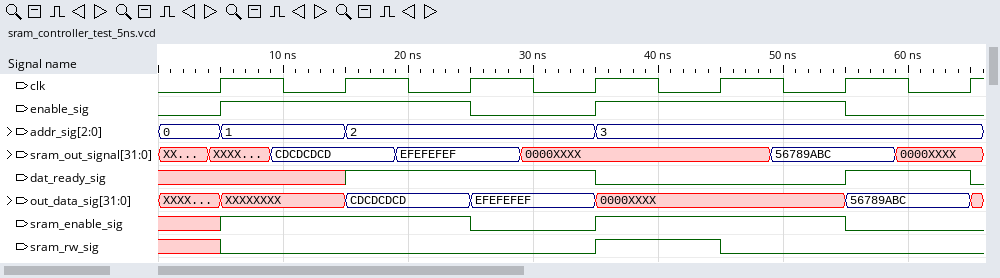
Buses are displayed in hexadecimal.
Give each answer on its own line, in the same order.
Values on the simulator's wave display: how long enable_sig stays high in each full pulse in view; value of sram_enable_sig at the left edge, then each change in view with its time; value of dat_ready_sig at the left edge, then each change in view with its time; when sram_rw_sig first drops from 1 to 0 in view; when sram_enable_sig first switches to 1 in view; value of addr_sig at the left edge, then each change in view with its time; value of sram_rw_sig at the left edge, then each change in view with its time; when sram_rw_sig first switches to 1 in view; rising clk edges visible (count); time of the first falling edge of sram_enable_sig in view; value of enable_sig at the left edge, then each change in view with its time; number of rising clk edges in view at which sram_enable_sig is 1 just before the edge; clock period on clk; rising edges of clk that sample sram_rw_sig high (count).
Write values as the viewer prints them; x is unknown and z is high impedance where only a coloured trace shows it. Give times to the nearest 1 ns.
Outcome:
20 ns, 20 ns
x, 1 at 5 ns, 0 at 25 ns, 1 at 35 ns, 0 at 55 ns
x, 1 at 15 ns, 0 at 35 ns, 1 at 55 ns, 0 at 65 ns
45 ns
5 ns
0, 1 at 5 ns, 2 at 15 ns, 3 at 35 ns
x, 0 at 5 ns, 1 at 35 ns, 0 at 45 ns
35 ns
7
25 ns
0, 1 at 5 ns, 0 at 25 ns, 1 at 35 ns, 0 at 55 ns
4
10 ns
1
